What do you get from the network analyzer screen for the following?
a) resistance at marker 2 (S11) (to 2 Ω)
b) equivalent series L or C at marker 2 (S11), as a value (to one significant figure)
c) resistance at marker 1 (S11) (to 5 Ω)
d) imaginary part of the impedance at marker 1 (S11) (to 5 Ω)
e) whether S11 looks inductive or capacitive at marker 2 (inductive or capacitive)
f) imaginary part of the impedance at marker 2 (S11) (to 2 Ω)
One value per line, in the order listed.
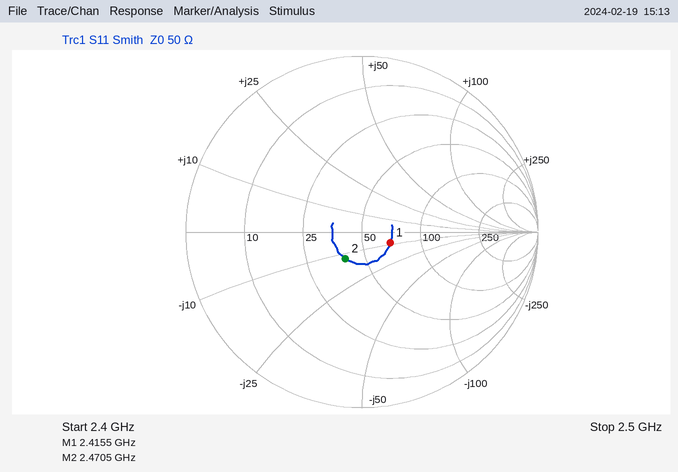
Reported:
40 Ω
5 pF
70 Ω
-10 Ω
capacitive
-12 Ω
